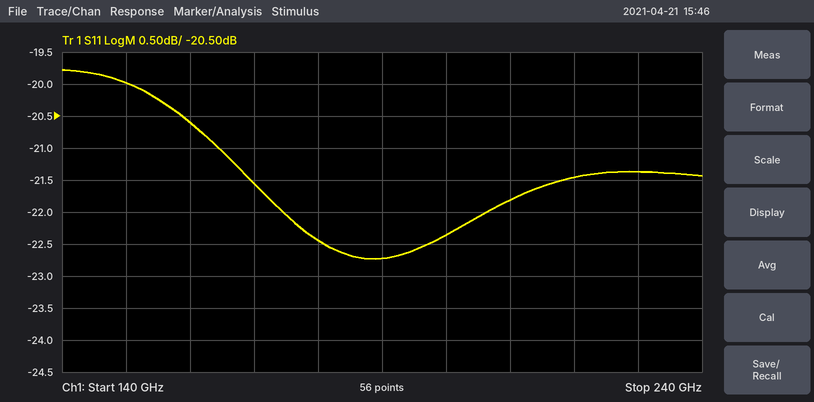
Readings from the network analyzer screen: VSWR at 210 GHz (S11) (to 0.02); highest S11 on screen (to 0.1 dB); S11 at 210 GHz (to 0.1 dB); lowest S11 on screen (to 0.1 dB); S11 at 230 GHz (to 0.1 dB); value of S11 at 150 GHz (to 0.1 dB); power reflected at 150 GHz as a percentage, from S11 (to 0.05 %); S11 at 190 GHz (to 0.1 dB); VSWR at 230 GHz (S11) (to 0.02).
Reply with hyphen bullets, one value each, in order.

- 1.18
- -19.8 dB
- -21.8 dB
- -22.7 dB
- -21.4 dB
- -20.0 dB
- 1.00 %
- -22.7 dB
- 1.18
